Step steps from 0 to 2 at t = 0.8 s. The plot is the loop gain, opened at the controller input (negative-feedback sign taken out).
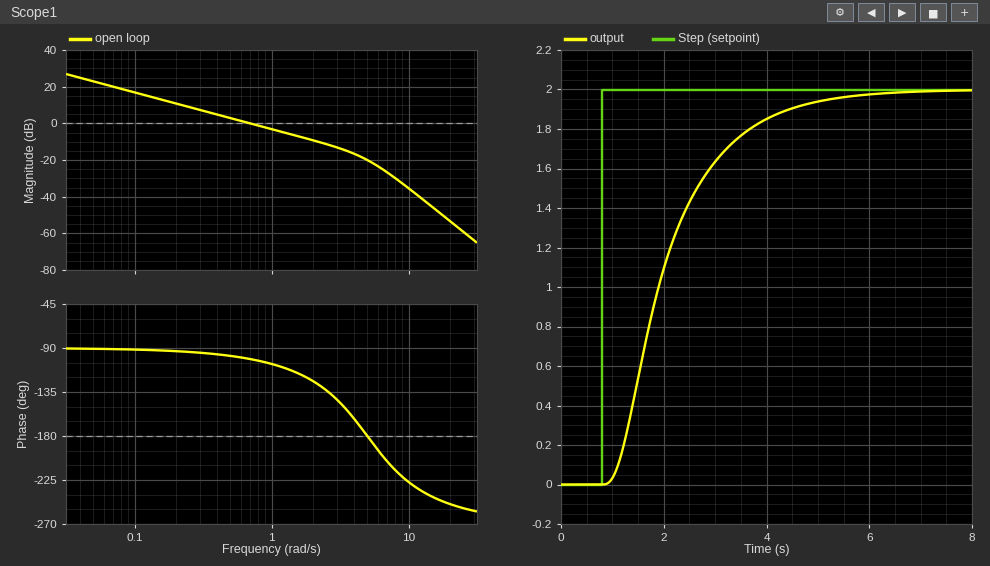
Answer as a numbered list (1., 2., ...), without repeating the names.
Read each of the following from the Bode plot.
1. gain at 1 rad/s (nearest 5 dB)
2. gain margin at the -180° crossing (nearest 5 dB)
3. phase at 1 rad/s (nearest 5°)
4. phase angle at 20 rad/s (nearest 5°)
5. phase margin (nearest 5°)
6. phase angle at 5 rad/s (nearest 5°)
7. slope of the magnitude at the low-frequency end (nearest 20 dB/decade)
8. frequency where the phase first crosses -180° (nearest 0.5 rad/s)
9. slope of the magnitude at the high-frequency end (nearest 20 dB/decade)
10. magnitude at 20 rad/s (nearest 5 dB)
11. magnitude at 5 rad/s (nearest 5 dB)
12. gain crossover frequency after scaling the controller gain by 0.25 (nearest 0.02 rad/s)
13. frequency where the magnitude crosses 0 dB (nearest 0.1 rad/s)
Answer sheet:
1. -5 dB
2. 20 dB
3. -105°
4. -250°
5. 80°
6. -180°
7. -20 dB/decade
8. 5.0 rad/s
9. -60 dB/decade
10. -55 dB
11. -20 dB
12. 0.18 rad/s
13. 0.7 rad/s
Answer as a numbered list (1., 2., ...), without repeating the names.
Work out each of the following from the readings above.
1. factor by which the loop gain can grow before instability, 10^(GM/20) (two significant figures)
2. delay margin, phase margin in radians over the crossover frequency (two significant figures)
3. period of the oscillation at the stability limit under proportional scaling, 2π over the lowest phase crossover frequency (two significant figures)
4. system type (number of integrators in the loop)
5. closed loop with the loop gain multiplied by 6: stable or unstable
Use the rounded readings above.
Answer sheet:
1. 10
2. 2.0 s
3. 1.3 s
4. 1
5. stable
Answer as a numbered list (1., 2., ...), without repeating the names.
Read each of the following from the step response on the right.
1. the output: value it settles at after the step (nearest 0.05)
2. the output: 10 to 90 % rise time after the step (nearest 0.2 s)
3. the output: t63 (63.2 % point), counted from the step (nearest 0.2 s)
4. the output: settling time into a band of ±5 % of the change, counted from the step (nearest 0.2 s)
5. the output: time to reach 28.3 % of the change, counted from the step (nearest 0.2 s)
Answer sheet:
1. 2.00
2. 2.4 s
3. 1.4 s
4. 3.6 s
5. 0.8 s
